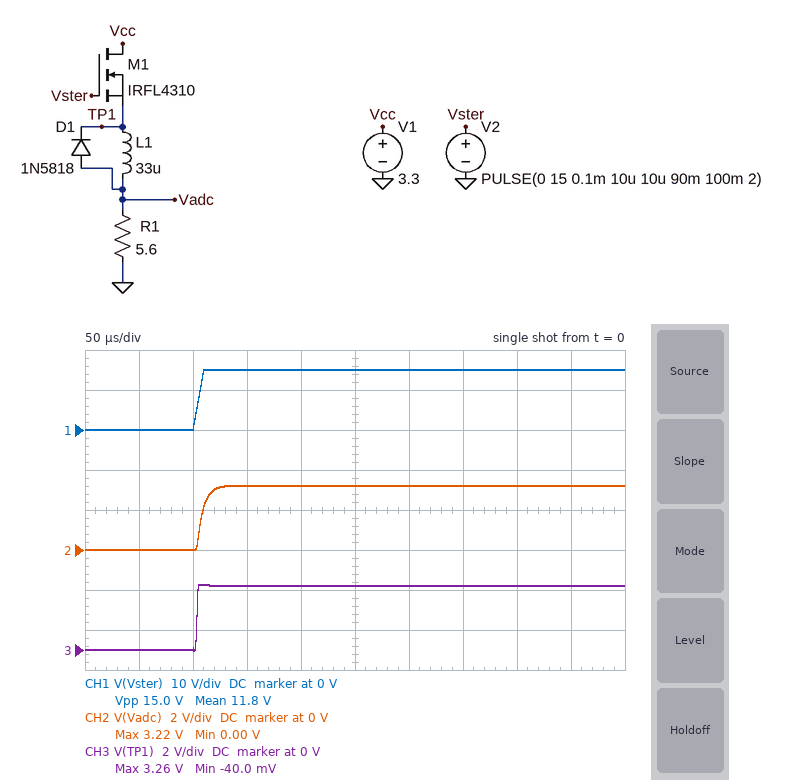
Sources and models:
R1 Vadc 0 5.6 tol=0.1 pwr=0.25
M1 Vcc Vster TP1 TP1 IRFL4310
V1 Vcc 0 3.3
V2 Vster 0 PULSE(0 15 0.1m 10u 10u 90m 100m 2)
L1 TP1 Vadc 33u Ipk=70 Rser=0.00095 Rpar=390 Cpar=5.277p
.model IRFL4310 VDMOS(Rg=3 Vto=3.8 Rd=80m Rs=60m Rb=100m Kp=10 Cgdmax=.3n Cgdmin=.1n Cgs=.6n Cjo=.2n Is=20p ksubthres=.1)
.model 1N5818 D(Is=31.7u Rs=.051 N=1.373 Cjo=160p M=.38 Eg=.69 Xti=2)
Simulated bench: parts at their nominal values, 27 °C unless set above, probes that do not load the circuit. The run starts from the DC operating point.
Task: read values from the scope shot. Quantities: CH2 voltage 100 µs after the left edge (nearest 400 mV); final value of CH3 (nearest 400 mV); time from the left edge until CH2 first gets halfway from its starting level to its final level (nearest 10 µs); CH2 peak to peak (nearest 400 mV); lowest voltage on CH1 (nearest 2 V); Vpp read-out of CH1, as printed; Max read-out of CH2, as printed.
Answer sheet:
0 V
3.2 V
110 µs
3.2 V
0 V
15.0 V
3.22 V
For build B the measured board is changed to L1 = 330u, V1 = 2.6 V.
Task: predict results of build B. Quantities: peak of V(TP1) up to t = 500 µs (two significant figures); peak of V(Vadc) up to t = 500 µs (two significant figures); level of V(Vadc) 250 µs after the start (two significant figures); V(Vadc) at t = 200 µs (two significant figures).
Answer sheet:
2.6 V
2.5 V
2.3 V
2.1 V
